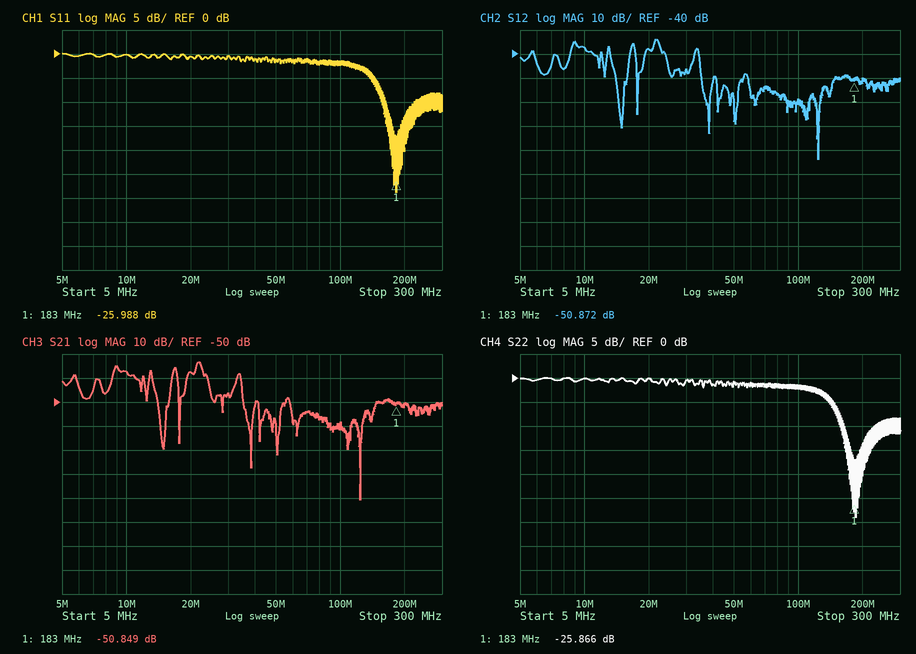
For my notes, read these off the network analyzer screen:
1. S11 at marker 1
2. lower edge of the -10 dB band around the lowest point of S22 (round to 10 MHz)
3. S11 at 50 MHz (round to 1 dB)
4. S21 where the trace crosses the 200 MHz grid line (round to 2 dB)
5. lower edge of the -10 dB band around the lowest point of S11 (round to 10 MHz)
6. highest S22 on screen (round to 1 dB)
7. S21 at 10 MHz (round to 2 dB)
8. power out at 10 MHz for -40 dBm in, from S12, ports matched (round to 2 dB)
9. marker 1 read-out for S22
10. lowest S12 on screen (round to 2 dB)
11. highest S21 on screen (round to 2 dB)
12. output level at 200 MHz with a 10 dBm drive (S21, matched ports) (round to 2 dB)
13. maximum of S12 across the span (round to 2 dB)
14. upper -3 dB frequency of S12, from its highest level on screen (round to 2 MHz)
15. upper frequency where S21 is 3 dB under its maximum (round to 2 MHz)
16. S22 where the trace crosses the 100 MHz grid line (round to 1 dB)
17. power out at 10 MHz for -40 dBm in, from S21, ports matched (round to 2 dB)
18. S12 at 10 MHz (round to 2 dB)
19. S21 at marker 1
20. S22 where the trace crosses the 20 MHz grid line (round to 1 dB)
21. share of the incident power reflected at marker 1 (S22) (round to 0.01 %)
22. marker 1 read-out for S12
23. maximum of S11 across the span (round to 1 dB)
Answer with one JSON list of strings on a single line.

["-25.988 dB", "160 MHz", "-1 dB", "-52 dB", "160 MHz", "0 dB", "-38 dB", "-78 dBm", "-25.866 dB", "-84 dB", "-34 dB", "-42 dBm", "-34 dB", "22 MHz", "22 MHz", "-2 dB", "-78 dBm", "-38 dB", "-50.849 dB", "0 dB", "0.26 %", "-50.872 dB", "0 dB"]
